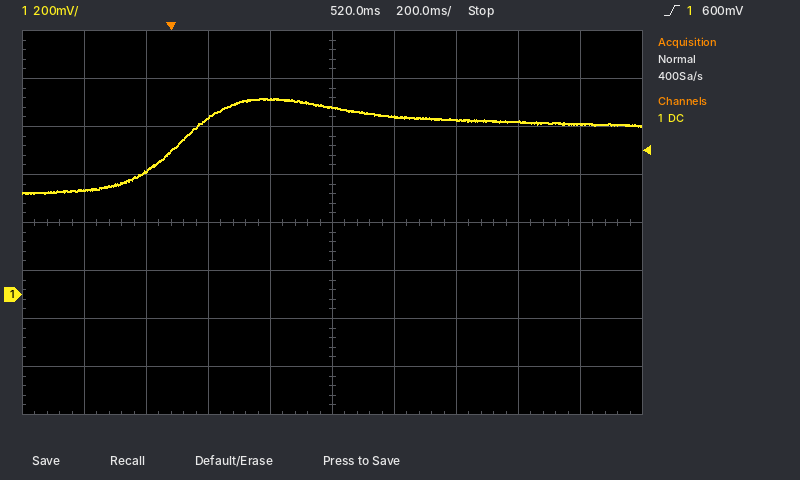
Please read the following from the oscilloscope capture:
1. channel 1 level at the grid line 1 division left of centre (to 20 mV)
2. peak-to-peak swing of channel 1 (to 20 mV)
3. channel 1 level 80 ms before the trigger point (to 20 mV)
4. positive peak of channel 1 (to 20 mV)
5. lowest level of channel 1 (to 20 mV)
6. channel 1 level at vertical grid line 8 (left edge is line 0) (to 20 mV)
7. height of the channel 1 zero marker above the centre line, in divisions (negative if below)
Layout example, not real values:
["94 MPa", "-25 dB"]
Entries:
["820 mV", "400 mV", "520 mV", "820 mV", "420 mV", "720 mV", "-1.5 div"]
